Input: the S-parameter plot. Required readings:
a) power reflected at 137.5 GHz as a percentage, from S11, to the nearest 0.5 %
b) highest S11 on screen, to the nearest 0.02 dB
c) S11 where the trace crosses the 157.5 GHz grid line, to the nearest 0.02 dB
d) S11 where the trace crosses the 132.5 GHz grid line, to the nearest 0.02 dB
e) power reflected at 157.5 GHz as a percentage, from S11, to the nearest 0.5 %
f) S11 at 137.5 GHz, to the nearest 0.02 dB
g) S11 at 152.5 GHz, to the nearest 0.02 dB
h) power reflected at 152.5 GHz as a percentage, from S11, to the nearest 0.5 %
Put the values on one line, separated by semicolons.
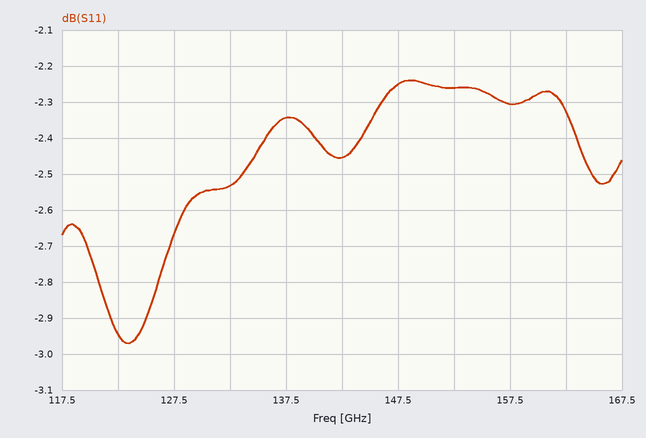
58.5 %; -2.24 dB; -2.30 dB; -2.54 dB; 59.0 %; -2.34 dB; -2.26 dB; 59.5 %
